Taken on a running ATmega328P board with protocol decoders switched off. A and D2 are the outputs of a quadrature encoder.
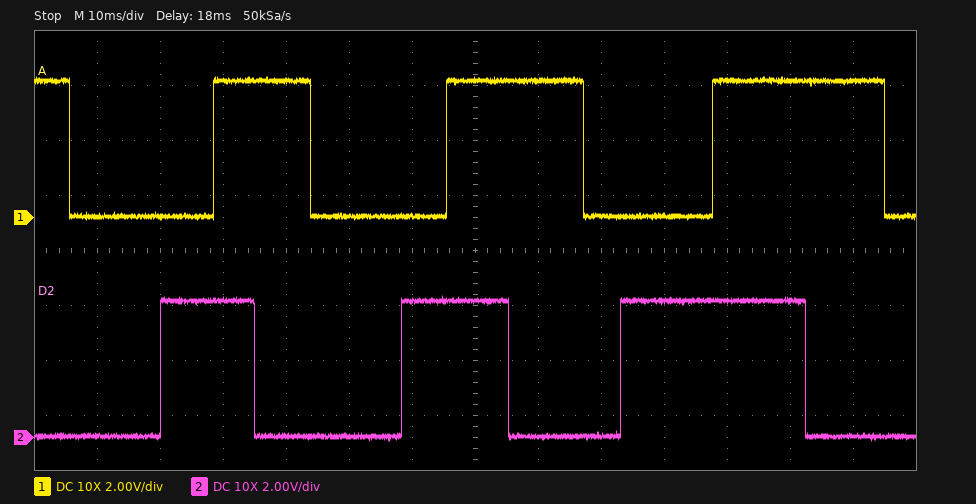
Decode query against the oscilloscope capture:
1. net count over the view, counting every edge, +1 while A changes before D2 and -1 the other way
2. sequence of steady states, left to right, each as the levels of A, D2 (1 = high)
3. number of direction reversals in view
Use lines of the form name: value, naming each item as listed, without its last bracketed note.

net count over the view, counting every edge, +1 while A changes before D2 and -1 the other way: -13
sequence of steady states, left to right, each as the levels of A, D2: 10 00 01 11 10 00 01 11 10 00 01 11 10 00
number of direction reversals in view: 0
